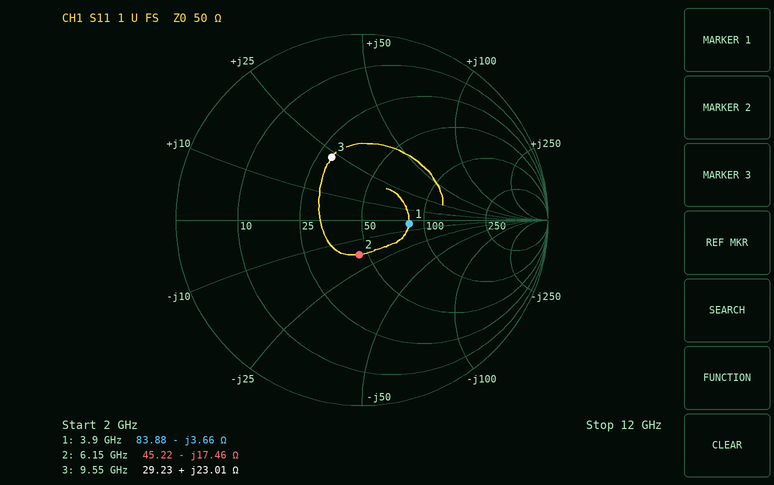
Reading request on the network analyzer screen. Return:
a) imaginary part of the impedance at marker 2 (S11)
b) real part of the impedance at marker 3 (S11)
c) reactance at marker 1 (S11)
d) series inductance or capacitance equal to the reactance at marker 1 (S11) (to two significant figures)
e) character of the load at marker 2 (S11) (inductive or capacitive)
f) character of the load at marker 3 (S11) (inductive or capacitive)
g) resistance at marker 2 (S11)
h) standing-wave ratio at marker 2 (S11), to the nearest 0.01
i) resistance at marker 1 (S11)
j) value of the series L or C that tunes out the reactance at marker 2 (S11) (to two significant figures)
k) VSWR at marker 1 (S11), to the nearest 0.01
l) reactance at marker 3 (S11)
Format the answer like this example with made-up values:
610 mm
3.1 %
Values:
-17.46 Ω
29.23 Ω
-3.66 Ω
11 pF
capacitive
inductive
45.22 Ω
1.46
83.88 Ω
450 pH
1.68
+23.01 Ω
